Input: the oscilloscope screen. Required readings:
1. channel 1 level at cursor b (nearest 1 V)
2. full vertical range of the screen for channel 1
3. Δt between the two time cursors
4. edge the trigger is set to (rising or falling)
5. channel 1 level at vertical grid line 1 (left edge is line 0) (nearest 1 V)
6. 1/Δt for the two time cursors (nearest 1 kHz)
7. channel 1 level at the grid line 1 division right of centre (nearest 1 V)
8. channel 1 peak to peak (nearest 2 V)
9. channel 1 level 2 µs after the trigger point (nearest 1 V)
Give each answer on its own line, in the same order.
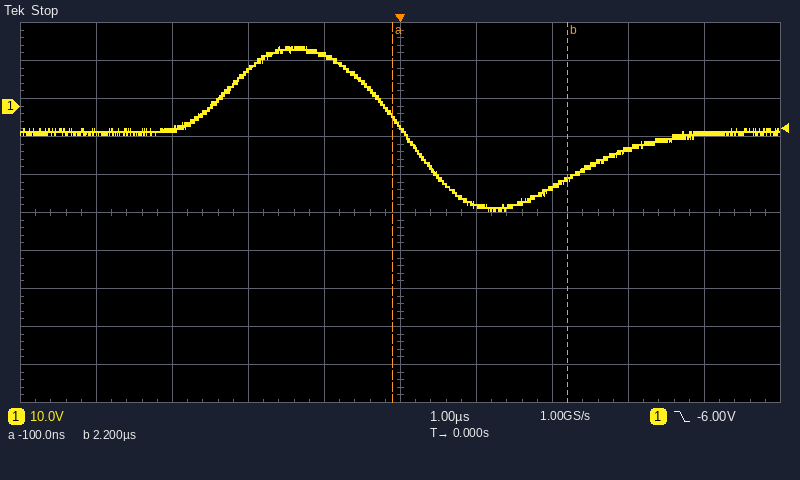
-19 V
100 V
2.3 µs
falling
-7 V
435 kHz
-26 V
44 V
-21 V
